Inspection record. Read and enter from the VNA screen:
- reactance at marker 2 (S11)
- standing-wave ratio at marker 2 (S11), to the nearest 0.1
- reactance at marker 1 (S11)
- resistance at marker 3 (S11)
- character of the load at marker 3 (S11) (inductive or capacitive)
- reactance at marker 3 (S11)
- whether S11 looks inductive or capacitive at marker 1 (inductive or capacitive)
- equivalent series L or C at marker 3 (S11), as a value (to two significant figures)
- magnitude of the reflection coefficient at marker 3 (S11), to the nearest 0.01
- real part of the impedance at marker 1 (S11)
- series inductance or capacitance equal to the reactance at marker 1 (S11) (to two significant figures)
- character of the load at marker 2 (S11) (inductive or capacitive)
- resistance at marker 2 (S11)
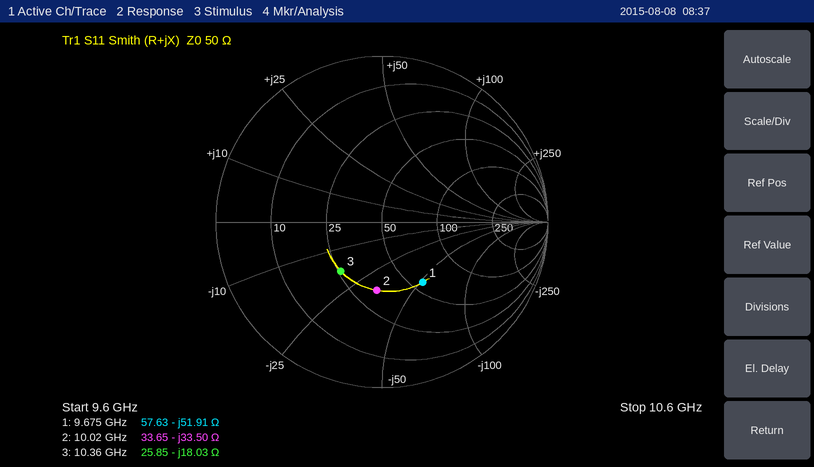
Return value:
-33.50 Ω
2.4
-51.91 Ω
25.85 Ω
capacitive
-18.03 Ω
capacitive
850 fF
0.39
57.63 Ω
320 fF
capacitive
33.65 Ω
